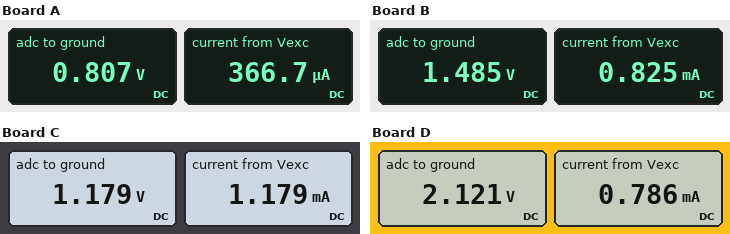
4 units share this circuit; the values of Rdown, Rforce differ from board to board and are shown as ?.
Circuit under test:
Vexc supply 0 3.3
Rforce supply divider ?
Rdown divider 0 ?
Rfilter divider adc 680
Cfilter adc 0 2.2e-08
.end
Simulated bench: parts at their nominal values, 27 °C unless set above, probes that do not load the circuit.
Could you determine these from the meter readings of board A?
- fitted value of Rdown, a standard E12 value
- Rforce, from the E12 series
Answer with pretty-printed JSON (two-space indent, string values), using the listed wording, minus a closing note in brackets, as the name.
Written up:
{
  "fitted value of Rdown, a standard E12 value": "2.2 kΩ",
  "Rforce, from the E12 series": "6.8 kΩ"
}
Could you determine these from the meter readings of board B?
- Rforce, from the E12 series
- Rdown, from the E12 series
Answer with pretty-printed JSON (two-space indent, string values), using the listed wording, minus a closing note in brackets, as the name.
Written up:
{
  "Rforce, from the E12 series": "2.2 kΩ",
  "Rdown, from the E12 series": "1.8 kΩ"
}
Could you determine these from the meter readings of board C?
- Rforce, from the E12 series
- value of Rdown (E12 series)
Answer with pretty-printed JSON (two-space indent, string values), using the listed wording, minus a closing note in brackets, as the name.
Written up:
{
  "Rforce, from the E12 series": "1.8 kΩ",
  "value of Rdown": "1 kΩ"
}
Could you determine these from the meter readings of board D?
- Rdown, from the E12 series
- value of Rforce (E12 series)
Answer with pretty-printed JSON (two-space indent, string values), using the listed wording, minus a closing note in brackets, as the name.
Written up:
{
  "Rdown, from the E12 series": "2.7 kΩ",
  "value of Rforce": "1.5 kΩ"
}
